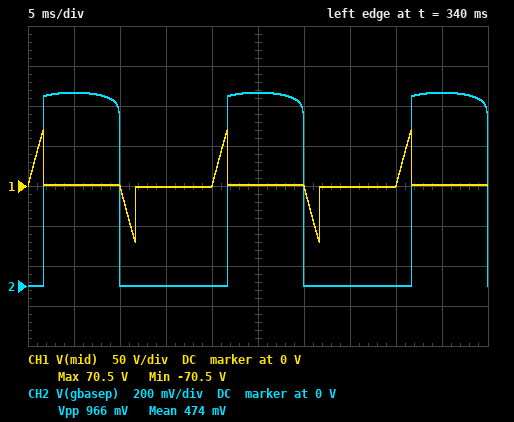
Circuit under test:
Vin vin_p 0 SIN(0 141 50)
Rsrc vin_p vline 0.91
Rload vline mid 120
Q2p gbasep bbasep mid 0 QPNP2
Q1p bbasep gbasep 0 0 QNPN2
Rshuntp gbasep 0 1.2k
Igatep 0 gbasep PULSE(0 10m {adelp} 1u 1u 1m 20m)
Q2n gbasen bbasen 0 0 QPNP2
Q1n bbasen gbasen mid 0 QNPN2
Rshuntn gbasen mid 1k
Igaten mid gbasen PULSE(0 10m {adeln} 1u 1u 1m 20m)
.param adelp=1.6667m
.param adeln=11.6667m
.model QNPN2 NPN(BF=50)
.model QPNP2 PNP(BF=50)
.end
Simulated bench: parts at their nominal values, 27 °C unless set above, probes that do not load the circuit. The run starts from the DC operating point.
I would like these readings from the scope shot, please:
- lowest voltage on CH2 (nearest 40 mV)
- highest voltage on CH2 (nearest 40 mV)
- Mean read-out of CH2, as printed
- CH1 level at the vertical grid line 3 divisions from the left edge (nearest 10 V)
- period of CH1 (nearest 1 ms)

0 V
960 mV
474 mV
0 V
20 ms
